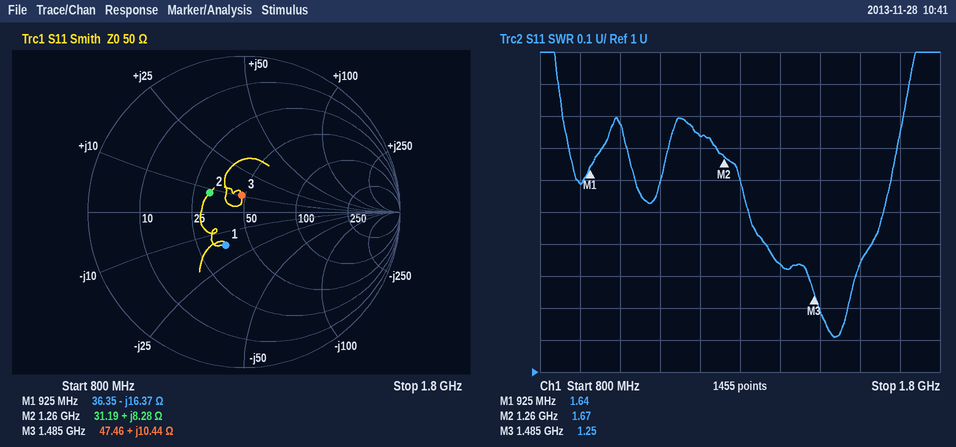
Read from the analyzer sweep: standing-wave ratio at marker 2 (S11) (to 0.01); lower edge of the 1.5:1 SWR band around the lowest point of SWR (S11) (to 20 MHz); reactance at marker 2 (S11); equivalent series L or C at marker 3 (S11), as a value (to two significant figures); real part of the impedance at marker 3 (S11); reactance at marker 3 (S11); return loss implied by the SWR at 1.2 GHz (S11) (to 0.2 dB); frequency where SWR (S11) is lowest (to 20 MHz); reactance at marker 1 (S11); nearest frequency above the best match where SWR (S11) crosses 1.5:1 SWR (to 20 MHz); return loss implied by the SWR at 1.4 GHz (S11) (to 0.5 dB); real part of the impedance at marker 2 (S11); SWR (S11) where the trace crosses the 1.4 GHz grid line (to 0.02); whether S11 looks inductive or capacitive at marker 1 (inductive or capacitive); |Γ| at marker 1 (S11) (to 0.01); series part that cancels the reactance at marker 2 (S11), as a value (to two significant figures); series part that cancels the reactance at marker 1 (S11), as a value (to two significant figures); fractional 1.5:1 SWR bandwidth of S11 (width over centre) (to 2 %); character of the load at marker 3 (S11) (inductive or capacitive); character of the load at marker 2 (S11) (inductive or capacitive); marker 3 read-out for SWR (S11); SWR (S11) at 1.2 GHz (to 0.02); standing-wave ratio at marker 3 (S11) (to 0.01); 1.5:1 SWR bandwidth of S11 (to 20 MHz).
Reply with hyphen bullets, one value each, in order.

- 1.67
- 1.32 GHz
- +8.28 Ω
- 1.1 nH
- 47.46 Ω
- +10.44 Ω
- 11.4 dB
- 1.54 GHz
- -16.37 Ω
- 1.66 GHz
- 17.0 dB
- 31.19 Ω
- 1.34
- capacitive
- 0.24
- 15 pF
- 2.8 nH
- 22 %
- inductive
- inductive
- 1.25
- 1.74
- 1.25
- 340 MHz
